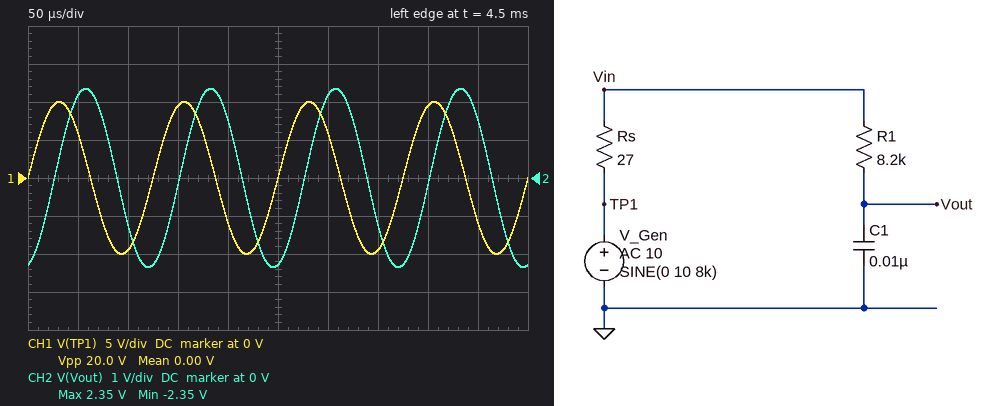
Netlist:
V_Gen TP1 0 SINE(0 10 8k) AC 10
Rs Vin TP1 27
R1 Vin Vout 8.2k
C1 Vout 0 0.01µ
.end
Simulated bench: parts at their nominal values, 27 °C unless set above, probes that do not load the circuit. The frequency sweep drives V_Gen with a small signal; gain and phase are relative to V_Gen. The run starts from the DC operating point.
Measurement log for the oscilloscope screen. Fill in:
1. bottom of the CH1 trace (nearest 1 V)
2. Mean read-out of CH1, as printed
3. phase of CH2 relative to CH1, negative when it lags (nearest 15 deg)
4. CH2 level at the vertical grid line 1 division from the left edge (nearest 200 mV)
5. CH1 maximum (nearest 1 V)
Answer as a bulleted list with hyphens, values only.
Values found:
- -10 V
- 0.00 V
- -75 deg
- 2.2 V
- 10 V
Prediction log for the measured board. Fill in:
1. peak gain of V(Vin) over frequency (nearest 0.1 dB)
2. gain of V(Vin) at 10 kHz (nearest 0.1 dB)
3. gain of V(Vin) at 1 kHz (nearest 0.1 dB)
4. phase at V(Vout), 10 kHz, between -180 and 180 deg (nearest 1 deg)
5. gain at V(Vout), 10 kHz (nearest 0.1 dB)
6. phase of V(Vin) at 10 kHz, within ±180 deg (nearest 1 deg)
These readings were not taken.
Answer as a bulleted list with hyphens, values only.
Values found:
- 0 dB
- 0 dB
- 0 dB
- -79 deg
- -14.4 dB
- 0 deg
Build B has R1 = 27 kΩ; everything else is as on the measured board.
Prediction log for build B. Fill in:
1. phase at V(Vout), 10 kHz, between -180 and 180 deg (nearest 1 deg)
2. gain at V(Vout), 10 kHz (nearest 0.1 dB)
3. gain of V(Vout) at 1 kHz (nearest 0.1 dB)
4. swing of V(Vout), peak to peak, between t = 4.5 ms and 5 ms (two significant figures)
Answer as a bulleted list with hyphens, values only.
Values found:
- -87 deg
- -24.6 dB
- -5.9 dB
- 1.5 V
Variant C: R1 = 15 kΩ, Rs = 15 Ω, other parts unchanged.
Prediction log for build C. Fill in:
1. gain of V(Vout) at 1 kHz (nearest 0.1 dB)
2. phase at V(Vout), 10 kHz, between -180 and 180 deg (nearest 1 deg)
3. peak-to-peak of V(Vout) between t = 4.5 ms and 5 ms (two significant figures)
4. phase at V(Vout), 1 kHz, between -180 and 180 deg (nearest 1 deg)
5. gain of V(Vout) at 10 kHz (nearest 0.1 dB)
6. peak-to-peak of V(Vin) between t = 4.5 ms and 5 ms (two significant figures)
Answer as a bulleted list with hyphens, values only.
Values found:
- -2.8 dB
- -84 deg
- 2.6 V
- -43 deg
- -19.5 dB
- 20 V
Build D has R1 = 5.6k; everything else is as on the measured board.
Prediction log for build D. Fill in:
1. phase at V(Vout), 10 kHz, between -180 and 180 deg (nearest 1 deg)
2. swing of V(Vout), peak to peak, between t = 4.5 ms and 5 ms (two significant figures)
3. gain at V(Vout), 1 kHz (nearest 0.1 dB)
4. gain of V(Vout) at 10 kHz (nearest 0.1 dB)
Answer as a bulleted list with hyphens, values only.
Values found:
- -74 deg
- 6.7 V
- -0.5 dB
- -11.3 dB
